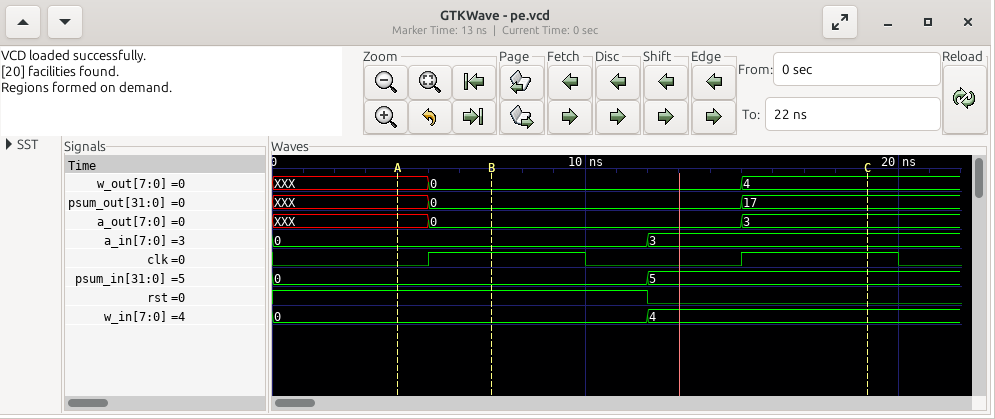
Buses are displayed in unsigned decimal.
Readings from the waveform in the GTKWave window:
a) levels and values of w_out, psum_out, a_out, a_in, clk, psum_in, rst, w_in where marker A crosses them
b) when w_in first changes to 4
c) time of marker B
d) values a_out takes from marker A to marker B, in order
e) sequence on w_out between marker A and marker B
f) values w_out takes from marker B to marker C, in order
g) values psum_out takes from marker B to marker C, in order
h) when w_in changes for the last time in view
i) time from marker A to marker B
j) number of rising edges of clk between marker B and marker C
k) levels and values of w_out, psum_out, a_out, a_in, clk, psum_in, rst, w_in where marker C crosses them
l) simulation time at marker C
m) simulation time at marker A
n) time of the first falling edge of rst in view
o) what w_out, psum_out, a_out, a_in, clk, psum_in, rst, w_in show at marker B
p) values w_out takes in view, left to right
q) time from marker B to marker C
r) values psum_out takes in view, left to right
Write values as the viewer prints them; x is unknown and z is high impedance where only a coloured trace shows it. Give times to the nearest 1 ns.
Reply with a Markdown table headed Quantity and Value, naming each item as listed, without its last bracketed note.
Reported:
| Quantity | Value |
|---|---|
| levels and values of w_out, psum_out, a_out, a_in, clk, psum_in, rst, w_in where marker A crosses them | w_out=XXX, psum_out=XXX, a_out=XXX, a_in=0, clk=0, psum_in=0, rst=1, w_in=0 |
| when w_in first changes to 4 | 12 ns |
| time of marker B | 7 ns |
| values a_out takes from marker A to marker B, in order | XXX, 0 |
| sequence on w_out between marker A and marker B | XXX, 0 |
| values w_out takes from marker B to marker C, in order | 0, 4 |
| values psum_out takes from marker B to marker C, in order | 0, 17 |
| when w_in changes for the last time in view | 12 ns |
| time from marker A to marker B | 3 ns |
| number of rising edges of clk between marker B and marker C | 1 |
| levels and values of w_out, psum_out, a_out, a_in, clk, psum_in, rst, w_in where marker C crosses them | w_out=4, psum_out=17, a_out=3, a_in=3, clk=1, psum_in=5, rst=0, w_in=4 |
| simulation time at marker C | 19 ns |
| simulation time at marker A | 4 ns |
| time of the first falling edge of rst in view | 12 ns |
| what w_out, psum_out, a_out, a_in, clk, psum_in, rst, w_in show at marker B | w_out=0, psum_out=0, a_out=0, a_in=0, clk=1, psum_in=0, rst=1, w_in=0 |
| values w_out takes in view, left to right | XXX, 0, 4 |
| time from marker B to marker C | 12 ns |
| values psum_out takes in view, left to right | XXX, 0, 17 |
